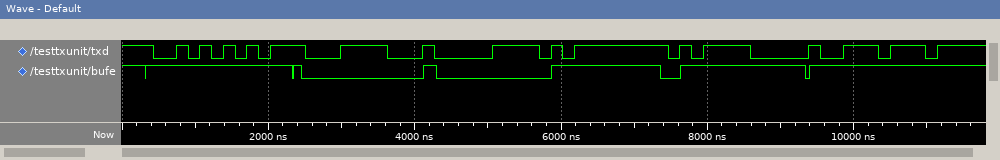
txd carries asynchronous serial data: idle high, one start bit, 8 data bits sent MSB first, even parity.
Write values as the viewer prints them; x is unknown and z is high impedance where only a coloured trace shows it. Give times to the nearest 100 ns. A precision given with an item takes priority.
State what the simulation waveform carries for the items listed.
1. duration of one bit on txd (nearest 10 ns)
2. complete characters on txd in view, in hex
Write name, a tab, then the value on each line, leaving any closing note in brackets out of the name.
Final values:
duration of one bit on txd	160 ns
complete characters on txd in view, in hex	55, 3C, 0F, FF, F0, 77
